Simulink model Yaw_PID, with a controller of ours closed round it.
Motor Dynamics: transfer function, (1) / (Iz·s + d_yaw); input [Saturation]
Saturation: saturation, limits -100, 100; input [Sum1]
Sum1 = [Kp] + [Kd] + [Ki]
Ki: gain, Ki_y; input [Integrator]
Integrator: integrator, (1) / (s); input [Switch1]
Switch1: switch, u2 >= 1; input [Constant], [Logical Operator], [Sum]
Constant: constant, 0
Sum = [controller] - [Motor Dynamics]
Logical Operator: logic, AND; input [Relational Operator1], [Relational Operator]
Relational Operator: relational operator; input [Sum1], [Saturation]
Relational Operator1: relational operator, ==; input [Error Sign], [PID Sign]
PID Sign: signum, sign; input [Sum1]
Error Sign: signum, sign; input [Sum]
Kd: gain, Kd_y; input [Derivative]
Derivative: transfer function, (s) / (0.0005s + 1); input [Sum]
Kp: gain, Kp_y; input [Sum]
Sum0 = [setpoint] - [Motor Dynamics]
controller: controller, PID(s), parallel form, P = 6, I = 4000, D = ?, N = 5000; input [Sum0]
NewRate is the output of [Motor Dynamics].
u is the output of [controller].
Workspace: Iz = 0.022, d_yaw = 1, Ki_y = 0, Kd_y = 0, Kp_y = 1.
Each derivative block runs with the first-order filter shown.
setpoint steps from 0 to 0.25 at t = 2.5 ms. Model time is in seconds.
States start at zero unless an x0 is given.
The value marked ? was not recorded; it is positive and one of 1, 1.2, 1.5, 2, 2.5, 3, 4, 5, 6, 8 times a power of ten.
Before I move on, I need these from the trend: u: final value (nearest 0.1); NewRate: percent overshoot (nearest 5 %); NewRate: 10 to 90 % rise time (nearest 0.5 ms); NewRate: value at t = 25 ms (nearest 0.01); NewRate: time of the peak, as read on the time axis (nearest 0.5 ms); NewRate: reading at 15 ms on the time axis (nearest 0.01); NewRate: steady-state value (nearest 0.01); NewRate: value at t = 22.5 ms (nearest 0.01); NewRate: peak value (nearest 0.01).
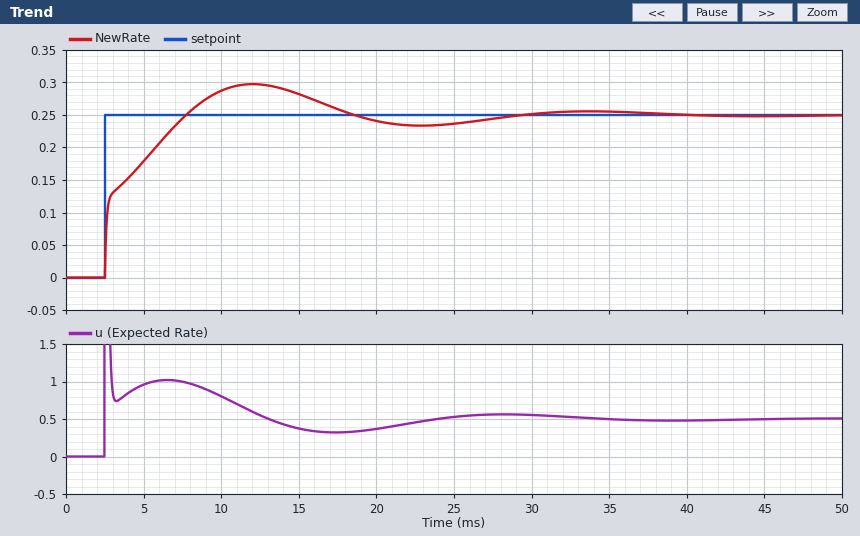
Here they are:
0.5
20 %
4.0 ms
0.24
12.0 ms
0.28
0.25
0.23
0.30
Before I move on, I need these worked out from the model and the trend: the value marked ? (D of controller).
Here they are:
0.02
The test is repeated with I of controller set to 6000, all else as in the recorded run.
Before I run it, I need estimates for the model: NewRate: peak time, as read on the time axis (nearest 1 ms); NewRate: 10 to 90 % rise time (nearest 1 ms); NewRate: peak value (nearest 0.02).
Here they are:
10 ms
3 ms
0.30
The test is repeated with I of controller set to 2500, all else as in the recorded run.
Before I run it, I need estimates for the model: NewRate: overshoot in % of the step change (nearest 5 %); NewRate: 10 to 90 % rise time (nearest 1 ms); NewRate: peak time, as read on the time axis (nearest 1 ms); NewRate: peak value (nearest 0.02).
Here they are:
15 %
5 ms
15 ms
0.28
